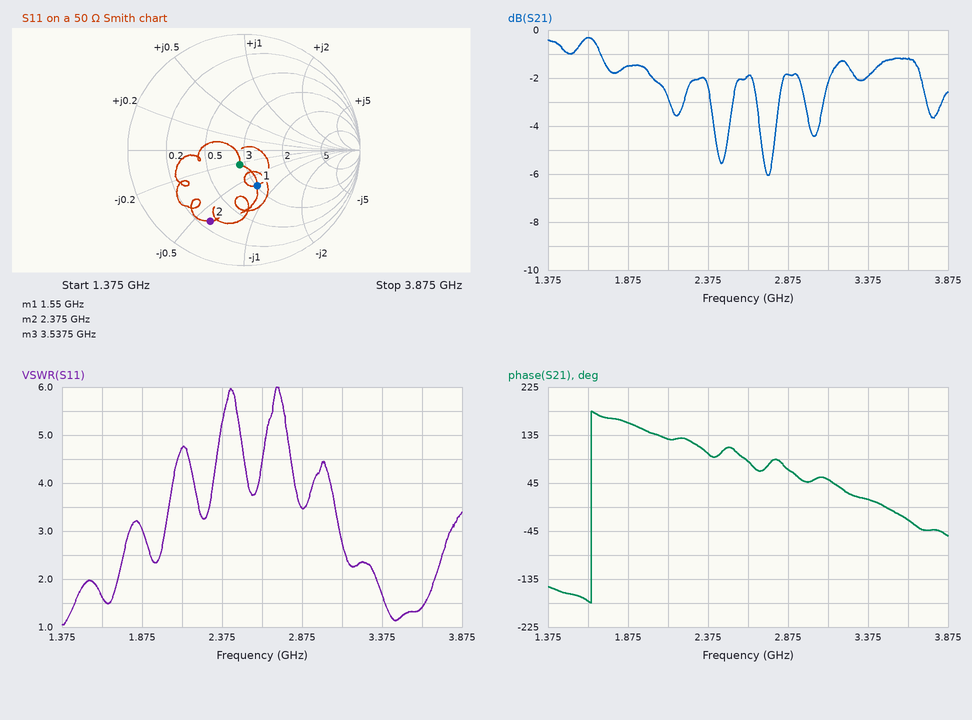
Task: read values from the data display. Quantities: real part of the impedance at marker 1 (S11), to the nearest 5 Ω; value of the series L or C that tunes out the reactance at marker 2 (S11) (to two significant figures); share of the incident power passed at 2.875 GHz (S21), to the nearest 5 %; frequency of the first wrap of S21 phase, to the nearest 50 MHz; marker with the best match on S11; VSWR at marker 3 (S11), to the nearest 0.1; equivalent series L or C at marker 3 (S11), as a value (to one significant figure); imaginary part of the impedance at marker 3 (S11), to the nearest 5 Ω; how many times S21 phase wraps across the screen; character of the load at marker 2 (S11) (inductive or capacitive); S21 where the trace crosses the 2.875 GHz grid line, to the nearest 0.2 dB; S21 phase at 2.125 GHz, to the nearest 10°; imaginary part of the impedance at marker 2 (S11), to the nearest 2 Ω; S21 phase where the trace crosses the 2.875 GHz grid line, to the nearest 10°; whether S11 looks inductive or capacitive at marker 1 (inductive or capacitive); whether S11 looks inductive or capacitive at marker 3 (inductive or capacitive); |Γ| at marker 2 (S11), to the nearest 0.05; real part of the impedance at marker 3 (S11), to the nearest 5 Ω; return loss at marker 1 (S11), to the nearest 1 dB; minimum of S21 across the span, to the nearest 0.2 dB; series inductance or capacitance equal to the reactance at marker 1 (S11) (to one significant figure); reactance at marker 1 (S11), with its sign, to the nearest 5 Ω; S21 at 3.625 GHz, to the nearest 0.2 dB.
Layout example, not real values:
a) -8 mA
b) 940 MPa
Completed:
a) 50 Ω
b) 2.0 nH
c) 65 %
d) 1.65 GHz
e) marker 3
f) 1.3
g) 4 pF
h) -10 Ω
i) 1
j) capacitive
k) -1.8 dB
l) 130°
m) -30 Ω
n) 70°
o) capacitive
p) capacitive
q) 0.70
r) 45 Ω
s) 10 dB
t) -6.0 dB
u) 3 pF
v) -35 Ω
w) -1.2 dB
